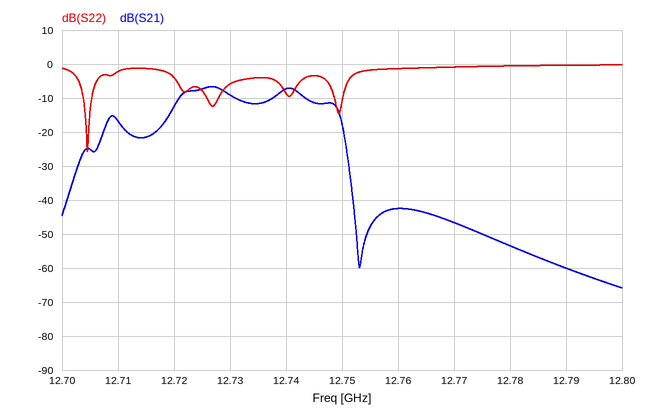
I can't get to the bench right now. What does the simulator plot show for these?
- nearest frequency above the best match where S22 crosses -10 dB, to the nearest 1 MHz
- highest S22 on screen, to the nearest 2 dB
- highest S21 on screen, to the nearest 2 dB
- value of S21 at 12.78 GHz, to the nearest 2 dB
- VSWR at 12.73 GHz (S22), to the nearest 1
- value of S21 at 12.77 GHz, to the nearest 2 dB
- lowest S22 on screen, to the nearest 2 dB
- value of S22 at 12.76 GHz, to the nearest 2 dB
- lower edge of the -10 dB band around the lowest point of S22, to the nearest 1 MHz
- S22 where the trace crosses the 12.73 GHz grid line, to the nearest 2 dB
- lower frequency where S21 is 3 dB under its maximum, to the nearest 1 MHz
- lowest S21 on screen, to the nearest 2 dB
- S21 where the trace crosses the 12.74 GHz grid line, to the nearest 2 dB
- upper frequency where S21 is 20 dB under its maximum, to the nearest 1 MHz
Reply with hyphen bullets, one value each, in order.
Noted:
- 12.705 GHz
- 0 dB
- -6 dB
- -54 dB
- 3
- -46 dB
- -26 dB
- -2 dB
- 12.704 GHz
- -6 dB
- 12.721 GHz
- -66 dB
- -8 dB
- 12.751 GHz
